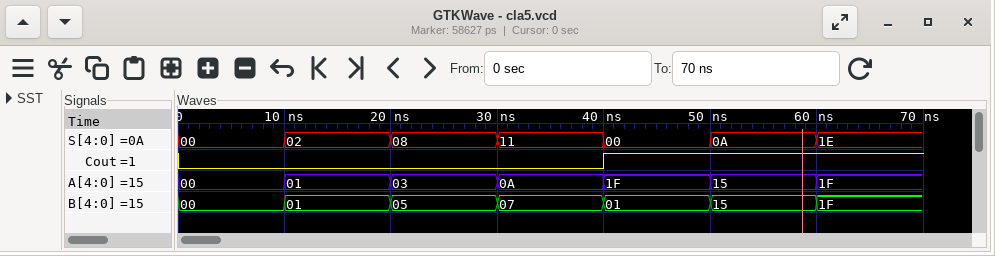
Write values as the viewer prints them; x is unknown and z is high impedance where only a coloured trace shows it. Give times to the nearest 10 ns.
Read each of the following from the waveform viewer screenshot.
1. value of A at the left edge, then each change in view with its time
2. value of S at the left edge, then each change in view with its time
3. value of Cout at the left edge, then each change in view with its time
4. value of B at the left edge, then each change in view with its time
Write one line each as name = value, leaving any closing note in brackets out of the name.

value of A at the left edge, then each change in view with its time = 00, 01 at 10 ns, 03 at 20 ns, 0A at 30 ns, 1F at 40 ns, 15 at 50 ns, 1F at 60 ns
value of S at the left edge, then each change in view with its time = 00, 02 at 10 ns, 08 at 20 ns, 11 at 30 ns, 00 at 40 ns, 0A at 50 ns, 1E at 60 ns
value of Cout at the left edge, then each change in view with its time = 0, 1 at 40 ns
value of B at the left edge, then each change in view with its time = 00, 01 at 10 ns, 05 at 20 ns, 07 at 30 ns, 01 at 40 ns, 15 at 50 ns, 1F at 60 ns
